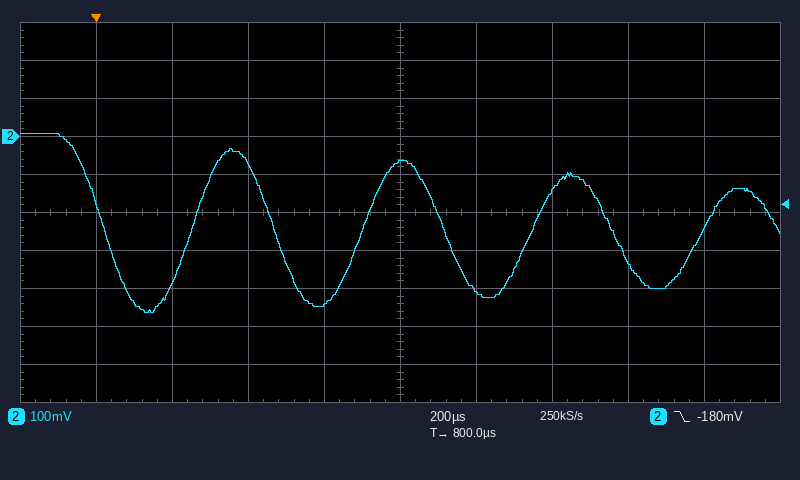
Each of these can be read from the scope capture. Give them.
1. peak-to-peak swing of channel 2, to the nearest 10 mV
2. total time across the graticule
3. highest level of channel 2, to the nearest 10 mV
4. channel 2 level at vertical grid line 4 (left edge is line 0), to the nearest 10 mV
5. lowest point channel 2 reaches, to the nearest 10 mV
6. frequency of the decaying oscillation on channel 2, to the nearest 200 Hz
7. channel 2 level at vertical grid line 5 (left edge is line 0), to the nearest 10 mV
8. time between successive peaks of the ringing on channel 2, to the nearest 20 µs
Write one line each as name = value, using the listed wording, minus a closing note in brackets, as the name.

peak-to-peak swing of channel 2, to the nearest 10 mV = 470 mV
total time across the graticule = 2 ms
highest level of channel 2, to the nearest 10 mV = 10 mV
channel 2 level at vertical grid line 4 (left edge is line 0), to the nearest 10 mV = -440 mV
lowest point channel 2 reaches, to the nearest 10 mV = -460 mV
frequency of the decaying oscillation on channel 2, to the nearest 200 Hz = 2.2 kHz
channel 2 level at vertical grid line 5 (left edge is line 0), to the nearest 10 mV = -70 mV
time between successive peaks of the ringing on channel 2, to the nearest 20 µs = 440 µs
